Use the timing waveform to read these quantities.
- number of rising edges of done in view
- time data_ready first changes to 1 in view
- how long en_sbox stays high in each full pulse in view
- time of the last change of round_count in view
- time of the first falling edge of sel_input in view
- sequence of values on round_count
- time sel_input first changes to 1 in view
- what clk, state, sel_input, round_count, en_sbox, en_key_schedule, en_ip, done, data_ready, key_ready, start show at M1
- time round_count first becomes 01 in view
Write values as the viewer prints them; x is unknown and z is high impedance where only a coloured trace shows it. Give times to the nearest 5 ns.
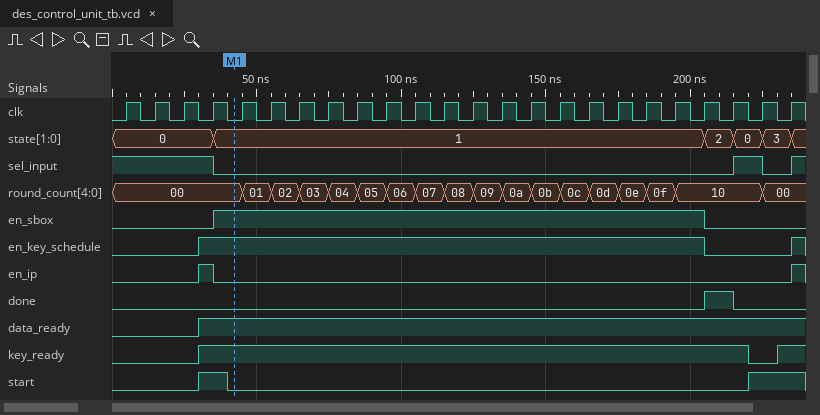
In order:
1
30 ns
170 ns
225 ns
35 ns
00, 01, 02, 03, 04, 05, 06, 07, 08, 09, 0a, 0b, 0c, 0d, 0e, 0f, 10, 00
215 ns
clk=0, state=1, sel_input=0, round_count=00, en_sbox=1, en_key_schedule=1, en_ip=0, done=0, data_ready=1, key_ready=1, start=0
45 ns
